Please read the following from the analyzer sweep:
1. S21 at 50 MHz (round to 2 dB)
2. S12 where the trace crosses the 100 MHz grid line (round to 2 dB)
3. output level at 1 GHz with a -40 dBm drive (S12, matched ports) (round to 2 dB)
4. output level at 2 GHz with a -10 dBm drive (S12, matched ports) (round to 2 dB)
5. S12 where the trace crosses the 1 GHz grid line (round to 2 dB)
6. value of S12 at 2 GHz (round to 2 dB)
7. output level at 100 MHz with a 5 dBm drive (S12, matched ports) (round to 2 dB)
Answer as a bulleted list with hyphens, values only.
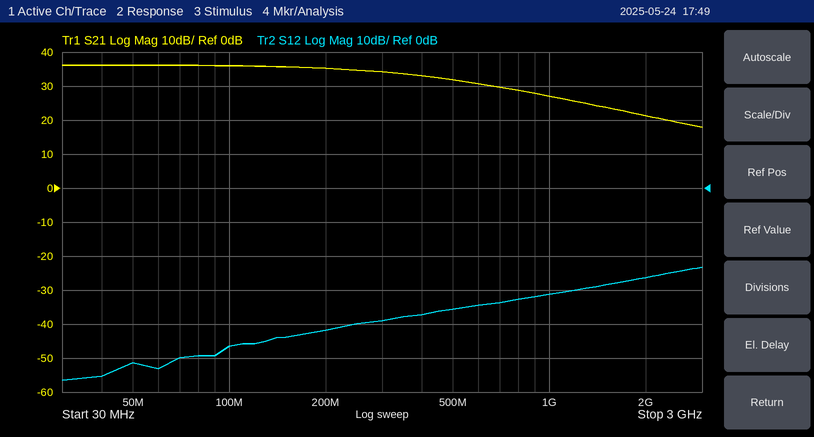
- 36 dB
- -46 dB
- -72 dBm
- -36 dBm
- -32 dB
- -26 dB
- -42 dBm
